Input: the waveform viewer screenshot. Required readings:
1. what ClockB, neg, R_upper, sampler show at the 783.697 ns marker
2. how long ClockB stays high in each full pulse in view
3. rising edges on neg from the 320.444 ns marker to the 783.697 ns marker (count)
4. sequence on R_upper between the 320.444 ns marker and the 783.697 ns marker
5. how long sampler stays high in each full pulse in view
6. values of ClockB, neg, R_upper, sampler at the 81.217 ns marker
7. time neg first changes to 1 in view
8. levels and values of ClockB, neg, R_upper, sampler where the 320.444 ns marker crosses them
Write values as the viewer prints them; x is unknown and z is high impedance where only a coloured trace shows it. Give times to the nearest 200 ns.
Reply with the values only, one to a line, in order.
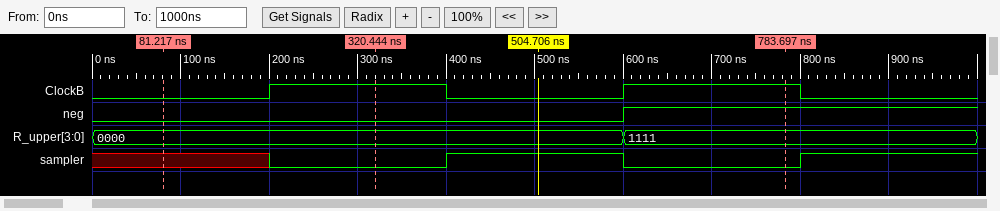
ClockB=1, neg=1, R_upper=1111, sampler=0
200 ns, 200 ns
1
0000, 1111
200 ns
ClockB=0, neg=0, R_upper=0000, sampler=x
600 ns
ClockB=1, neg=0, R_upper=0000, sampler=0
